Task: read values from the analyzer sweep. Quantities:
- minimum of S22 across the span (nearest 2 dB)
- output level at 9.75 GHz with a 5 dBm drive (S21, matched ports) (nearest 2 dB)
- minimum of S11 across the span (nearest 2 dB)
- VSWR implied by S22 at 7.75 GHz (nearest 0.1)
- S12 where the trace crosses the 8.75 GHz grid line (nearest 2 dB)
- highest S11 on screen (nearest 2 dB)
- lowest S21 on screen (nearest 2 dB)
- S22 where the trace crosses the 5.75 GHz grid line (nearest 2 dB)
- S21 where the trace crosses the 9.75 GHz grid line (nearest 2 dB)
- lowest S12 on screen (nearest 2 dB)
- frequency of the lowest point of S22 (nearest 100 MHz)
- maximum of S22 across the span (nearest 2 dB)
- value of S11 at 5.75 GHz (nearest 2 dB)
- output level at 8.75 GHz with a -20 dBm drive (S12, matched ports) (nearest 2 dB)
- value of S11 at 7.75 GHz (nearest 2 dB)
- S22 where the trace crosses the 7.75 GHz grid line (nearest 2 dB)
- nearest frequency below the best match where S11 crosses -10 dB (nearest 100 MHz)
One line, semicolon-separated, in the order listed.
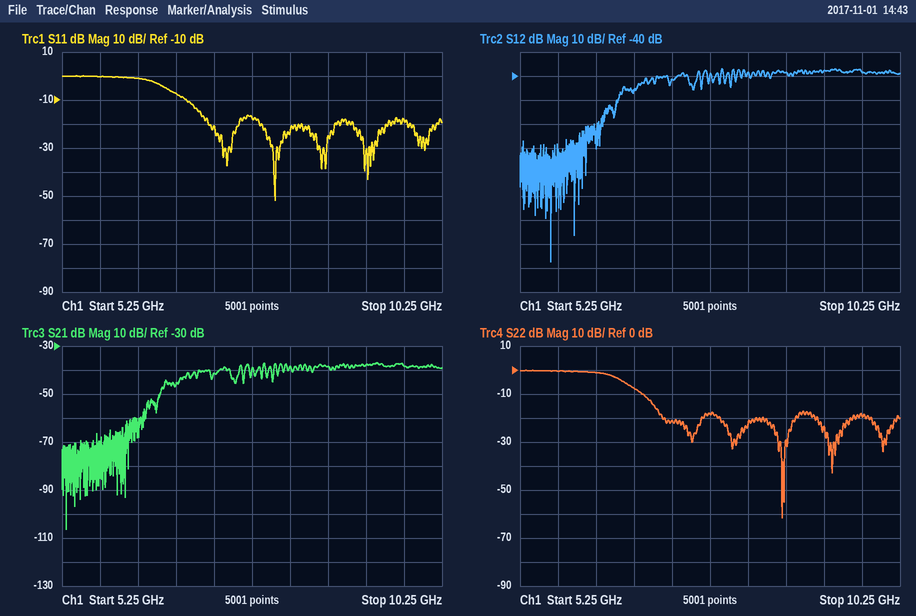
-62 dB; -34 dBm; -52 dB; 1.3; -38 dB; 0 dB; -106 dB; 0 dB; -38 dB; -118 dB; 8.7 GHz; 0 dB; 0 dB; -58 dBm; -18 dB; -18 dB; 6.9 GHz
